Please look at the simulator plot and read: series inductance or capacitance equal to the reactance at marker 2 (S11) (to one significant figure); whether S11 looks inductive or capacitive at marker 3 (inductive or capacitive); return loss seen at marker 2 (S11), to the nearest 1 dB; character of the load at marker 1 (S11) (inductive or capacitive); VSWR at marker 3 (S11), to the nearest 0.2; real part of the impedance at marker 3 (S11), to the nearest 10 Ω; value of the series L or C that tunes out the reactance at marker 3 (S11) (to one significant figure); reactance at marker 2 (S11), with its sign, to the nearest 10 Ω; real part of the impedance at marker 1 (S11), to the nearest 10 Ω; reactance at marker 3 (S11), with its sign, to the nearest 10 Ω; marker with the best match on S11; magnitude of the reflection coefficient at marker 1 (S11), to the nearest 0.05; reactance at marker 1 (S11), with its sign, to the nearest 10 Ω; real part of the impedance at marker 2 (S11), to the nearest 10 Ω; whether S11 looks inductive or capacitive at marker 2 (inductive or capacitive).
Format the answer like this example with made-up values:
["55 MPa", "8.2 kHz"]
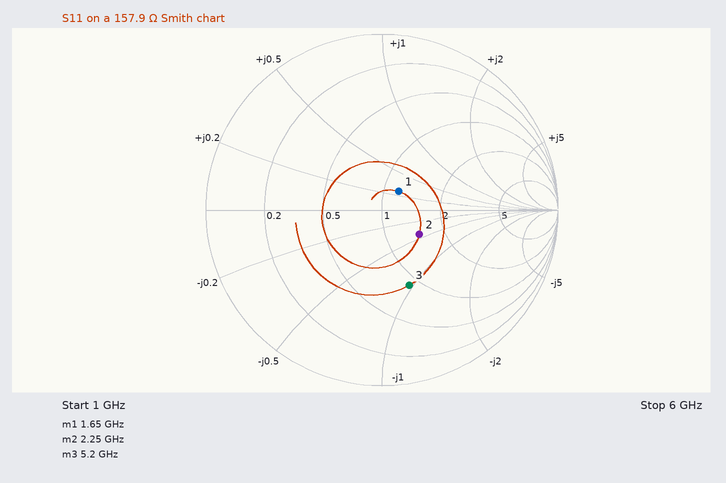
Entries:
["1 pF", "capacitive", "12 dB", "inductive", "2.6", "140 Ω", "5 nH", "-70 Ω", "190 Ω", "-150 Ω", "marker 1", "0.15", "+40 Ω", "230 Ω", "capacitive"]
